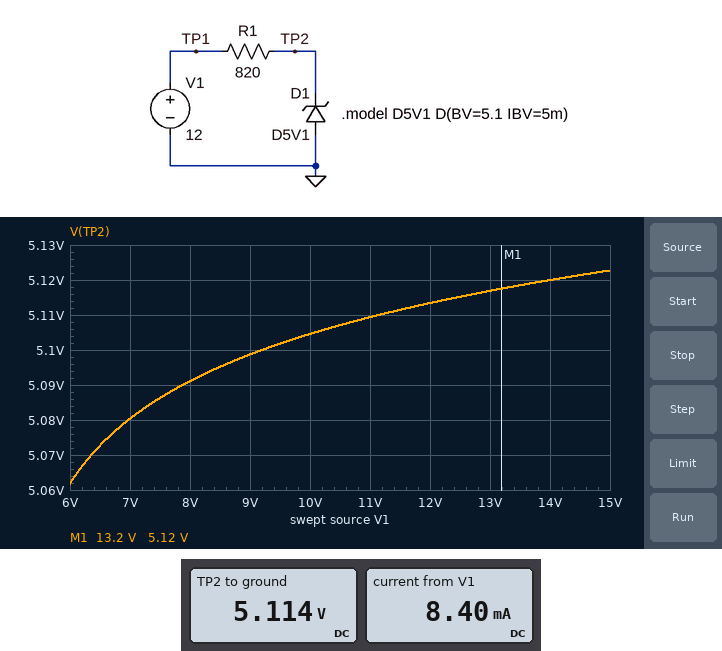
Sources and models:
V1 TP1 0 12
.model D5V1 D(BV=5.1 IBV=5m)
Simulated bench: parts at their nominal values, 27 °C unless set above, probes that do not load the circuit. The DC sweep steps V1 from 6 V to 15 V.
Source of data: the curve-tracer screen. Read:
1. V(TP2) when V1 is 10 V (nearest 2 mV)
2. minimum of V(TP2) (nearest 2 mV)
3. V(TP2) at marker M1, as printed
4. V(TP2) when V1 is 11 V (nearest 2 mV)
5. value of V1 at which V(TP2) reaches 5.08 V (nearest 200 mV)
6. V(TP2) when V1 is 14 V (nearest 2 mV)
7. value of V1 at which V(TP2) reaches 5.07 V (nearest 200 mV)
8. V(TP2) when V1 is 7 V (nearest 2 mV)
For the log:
5.104 V
5.062 V
5.12 V
5.110 V
7.0 V
5.120 V
6.4 V
5.080 V
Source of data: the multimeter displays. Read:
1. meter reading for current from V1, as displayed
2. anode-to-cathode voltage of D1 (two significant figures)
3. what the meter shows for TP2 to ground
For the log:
8.40 mA
-5.1 V
5.114 V
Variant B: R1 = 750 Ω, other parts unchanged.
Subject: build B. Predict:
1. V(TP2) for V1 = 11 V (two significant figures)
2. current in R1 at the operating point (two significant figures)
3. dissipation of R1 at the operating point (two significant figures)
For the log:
5.1 V
9.2 mA
63 mW
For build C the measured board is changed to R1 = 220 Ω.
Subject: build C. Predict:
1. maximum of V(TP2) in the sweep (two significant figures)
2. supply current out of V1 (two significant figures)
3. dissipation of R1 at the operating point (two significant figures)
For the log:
5.2 V
31 mA
210 mW
